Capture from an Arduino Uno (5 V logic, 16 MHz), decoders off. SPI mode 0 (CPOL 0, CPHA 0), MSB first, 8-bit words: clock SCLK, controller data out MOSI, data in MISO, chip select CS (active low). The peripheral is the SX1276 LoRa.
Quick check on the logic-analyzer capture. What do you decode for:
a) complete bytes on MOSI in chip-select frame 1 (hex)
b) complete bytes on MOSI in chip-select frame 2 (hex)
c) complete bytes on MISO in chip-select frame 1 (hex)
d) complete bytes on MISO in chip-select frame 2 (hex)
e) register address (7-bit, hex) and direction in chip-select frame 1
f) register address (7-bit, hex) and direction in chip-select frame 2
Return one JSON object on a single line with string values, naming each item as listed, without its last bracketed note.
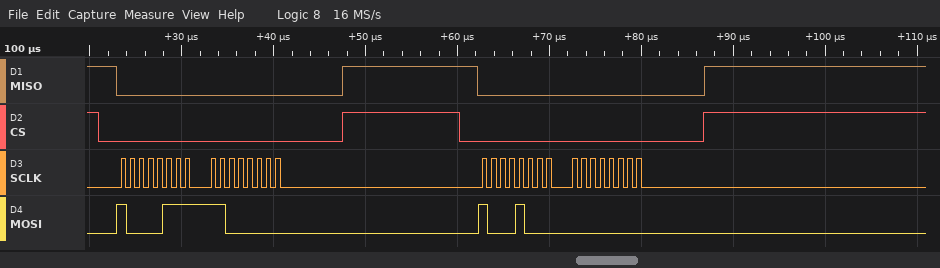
{"complete bytes on MOSI in chip-select frame 1": "87 C0", "complete bytes on MOSI in chip-select frame 2": "88 00", "complete bytes on MISO in chip-select frame 1": "00 00", "complete bytes on MISO in chip-select frame 2": "00 00", "register address (7-bit, hex) and direction in chip-select frame 1": "0x07 write", "register address (7-bit, hex) and direction in chip-select frame 2": "0x08 write"}
